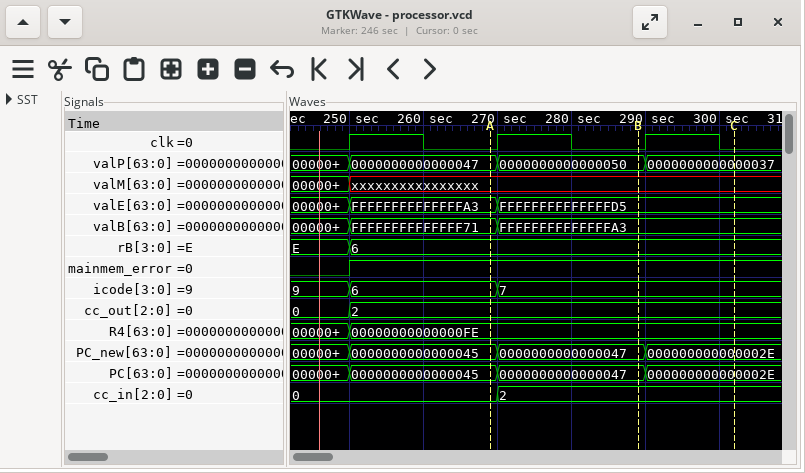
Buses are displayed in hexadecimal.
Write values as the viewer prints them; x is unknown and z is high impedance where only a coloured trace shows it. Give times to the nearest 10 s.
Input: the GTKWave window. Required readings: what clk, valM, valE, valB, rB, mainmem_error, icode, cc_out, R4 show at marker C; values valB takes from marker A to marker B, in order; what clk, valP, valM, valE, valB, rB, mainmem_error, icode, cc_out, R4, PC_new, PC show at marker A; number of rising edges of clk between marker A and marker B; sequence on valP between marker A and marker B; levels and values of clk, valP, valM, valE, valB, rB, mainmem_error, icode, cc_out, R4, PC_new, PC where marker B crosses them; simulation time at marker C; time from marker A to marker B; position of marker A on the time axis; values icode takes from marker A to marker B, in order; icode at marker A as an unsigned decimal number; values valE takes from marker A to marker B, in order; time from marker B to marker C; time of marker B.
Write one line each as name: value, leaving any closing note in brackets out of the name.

what clk, valM, valE, valB, rB, mainmem_error, icode, cc_out, R4 show at marker C: clk=0, valM=xxxxxxxxxxxxxxxx, valE=FFFFFFFFFFFFFFD5, valB=FFFFFFFFFFFFFFA3, rB=6, mainmem_error=1, icode=7, cc_out=2, R4=00000000000000FE
values valB takes from marker A to marker B, in order: FFFFFFFFFFFFFF71, FFFFFFFFFFFFFFA3
what clk, valP, valM, valE, valB, rB, mainmem_error, icode, cc_out, R4, PC_new, PC show at marker A: clk=0, valP=0000000000000047, valM=xxxxxxxxxxxxxxxx, valE=FFFFFFFFFFFFFFA3, valB=FFFFFFFFFFFFFF71, rB=6, mainmem_error=1, icode=6, cc_out=2, R4=00000000000000FE, PC_new=0000000000000045, PC=0000000000000045
number of rising edges of clk between marker A and marker B: 1
sequence on valP between marker A and marker B: 0000000000000047, 0000000000000050
levels and values of clk, valP, valM, valE, valB, rB, mainmem_error, icode, cc_out, R4, PC_new, PC where marker B crosses them: clk=0, valP=0000000000000050, valM=xxxxxxxxxxxxxxxx, valE=FFFFFFFFFFFFFFD5, valB=FFFFFFFFFFFFFFA3, rB=6, mainmem_error=1, icode=7, cc_out=2, R4=00000000000000FE, PC_new=0000000000000047, PC=0000000000000047
simulation time at marker C: 300 s
time from marker A to marker B: 20 s
position of marker A on the time axis: 270 s
values icode takes from marker A to marker B, in order: 6, 7
icode at marker A as an unsigned decimal number: 6
values valE takes from marker A to marker B, in order: FFFFFFFFFFFFFFA3, FFFFFFFFFFFFFFD5
time from marker B to marker C: 10 s
time of marker B: 290 s
